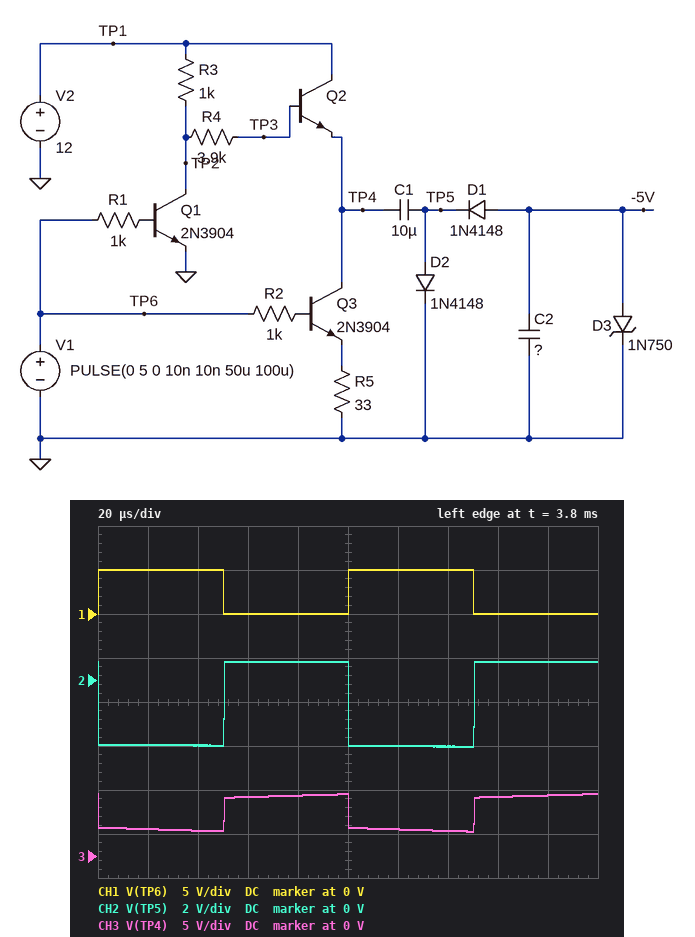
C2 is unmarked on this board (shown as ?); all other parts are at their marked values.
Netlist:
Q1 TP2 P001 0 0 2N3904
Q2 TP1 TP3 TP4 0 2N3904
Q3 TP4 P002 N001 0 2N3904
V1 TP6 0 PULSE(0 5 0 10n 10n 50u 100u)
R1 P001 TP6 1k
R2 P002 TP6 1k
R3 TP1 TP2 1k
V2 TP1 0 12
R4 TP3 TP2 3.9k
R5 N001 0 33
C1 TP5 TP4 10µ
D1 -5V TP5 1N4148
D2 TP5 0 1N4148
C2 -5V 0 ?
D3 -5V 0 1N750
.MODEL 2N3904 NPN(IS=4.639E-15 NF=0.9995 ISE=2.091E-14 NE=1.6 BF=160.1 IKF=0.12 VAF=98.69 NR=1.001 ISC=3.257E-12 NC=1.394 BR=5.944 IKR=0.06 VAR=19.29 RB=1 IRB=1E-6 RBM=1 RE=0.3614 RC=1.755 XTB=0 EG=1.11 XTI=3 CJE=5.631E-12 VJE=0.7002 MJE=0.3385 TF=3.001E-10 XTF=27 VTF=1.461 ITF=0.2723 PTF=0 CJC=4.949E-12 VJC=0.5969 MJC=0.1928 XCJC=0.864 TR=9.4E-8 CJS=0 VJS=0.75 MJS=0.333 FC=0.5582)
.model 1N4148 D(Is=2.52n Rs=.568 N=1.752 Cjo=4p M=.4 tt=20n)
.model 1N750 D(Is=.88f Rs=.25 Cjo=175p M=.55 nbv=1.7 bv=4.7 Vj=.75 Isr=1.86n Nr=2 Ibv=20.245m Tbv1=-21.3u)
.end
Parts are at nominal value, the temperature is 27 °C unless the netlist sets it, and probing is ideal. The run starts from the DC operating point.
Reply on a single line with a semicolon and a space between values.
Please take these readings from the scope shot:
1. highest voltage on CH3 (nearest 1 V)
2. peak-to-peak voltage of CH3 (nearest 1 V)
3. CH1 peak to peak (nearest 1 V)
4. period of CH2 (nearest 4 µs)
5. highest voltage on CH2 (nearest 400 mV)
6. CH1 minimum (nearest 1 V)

7 V; 4 V; 5 V; 100 µs; 800 mV; 0 V
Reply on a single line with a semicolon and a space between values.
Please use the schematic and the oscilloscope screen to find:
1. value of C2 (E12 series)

82 µF
